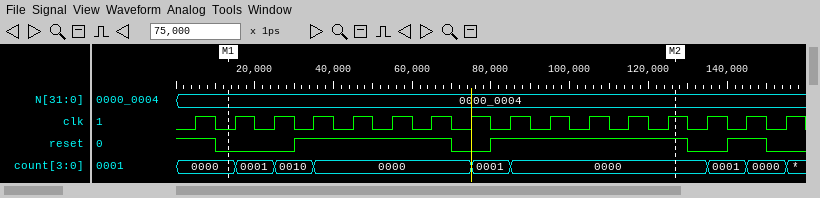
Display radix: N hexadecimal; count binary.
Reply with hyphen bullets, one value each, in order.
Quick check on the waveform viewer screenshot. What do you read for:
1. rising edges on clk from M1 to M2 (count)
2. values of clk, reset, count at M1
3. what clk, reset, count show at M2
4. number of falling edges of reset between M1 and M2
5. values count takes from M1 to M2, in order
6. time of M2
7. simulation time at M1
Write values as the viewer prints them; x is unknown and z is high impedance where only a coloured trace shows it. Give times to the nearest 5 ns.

- 12
- clk=0, reset=0, count=0000
- clk=1, reset=1, count=0000
- 1
- 0000, 0001, 0010, 0000, 0001, 0000
- 125 ns
- 15 ns
